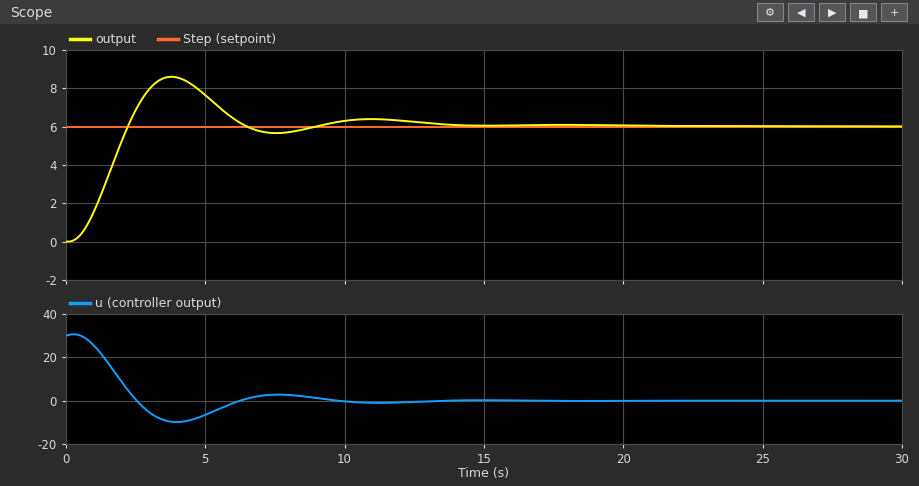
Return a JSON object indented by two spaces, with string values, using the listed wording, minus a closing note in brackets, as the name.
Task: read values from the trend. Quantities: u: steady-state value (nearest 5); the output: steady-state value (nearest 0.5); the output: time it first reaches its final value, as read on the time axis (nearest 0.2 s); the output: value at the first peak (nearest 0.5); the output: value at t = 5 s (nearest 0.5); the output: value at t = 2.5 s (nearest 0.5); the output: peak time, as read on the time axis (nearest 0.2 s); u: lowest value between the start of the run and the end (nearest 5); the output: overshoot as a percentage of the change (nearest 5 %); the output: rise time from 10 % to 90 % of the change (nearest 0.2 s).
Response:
{
  "u: steady-state value": "0",
  "the output: steady-state value": "6.0",
  "the output: time it first reaches its final value, as read on the time axis": "2.2 s",
  "the output: value at the first peak": "8.5",
  "the output: value at t = 5 s": "7.5",
  "the output: value at t = 2.5 s": "7.0",
  "the output: peak time, as read on the time axis": "3.8 s",
  "u: lowest value between the start of the run and the end": "-10",
  "the output: overshoot as a percentage of the change": "45 %",
  "the output: rise time from 10 % to 90 % of the change": "1.4 s"
}
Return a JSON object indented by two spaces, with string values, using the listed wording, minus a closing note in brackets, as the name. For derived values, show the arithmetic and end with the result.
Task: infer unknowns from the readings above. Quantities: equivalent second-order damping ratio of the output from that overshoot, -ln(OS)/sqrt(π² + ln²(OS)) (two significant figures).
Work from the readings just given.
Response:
{
  "equivalent second-order damping ratio of the output from that overshoot, -ln(OS)/sqrt(π² + ln²(OS))": "ln(0.45) = -0.799; 0.799 / sqrt(9.870 + 0.638) = 0.25"
}
